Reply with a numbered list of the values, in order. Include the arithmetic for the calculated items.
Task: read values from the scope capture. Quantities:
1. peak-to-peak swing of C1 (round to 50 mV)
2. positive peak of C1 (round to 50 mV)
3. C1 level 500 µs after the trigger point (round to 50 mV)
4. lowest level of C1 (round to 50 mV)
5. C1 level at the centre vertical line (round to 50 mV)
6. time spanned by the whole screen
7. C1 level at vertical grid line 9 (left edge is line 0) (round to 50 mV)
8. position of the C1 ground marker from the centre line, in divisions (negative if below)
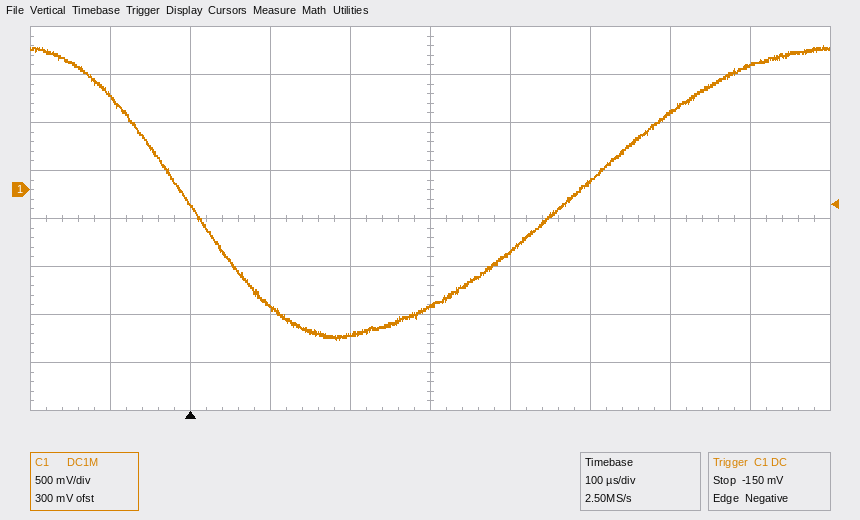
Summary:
1. 1.50 V − (-1.55 V) = 3.05 V
2. 1.50 V
3. 100 mV
4. -1.55 V
5. -1.20 V
6. 1 ms
7. 1.30 V
8. +0.6 div
